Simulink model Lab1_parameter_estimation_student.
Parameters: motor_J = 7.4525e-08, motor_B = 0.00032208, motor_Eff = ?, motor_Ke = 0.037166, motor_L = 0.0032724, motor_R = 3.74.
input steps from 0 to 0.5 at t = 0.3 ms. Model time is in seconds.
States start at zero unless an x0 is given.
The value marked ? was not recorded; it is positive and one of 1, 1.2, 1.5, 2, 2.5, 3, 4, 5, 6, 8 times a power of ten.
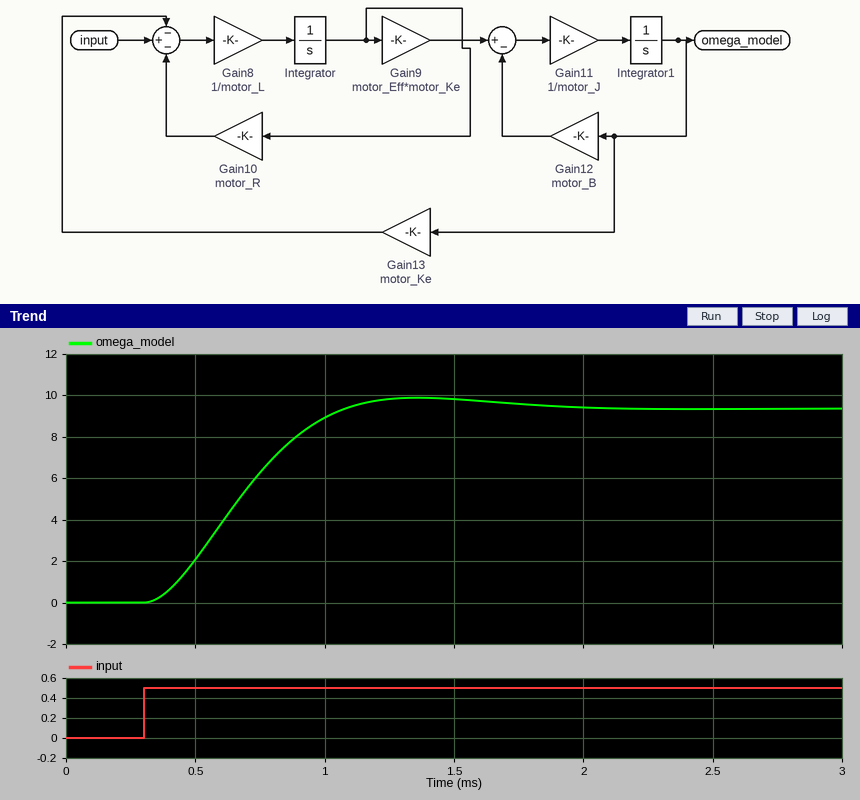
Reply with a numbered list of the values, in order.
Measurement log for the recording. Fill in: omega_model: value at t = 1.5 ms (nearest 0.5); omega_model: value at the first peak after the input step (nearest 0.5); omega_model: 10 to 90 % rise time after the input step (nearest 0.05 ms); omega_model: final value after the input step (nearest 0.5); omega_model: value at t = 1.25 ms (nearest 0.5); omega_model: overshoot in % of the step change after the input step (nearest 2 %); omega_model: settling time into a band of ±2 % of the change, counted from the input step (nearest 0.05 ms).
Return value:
1. 10.0
2. 10.0
3. 0.50 ms
4. 9.5
5. 10.0
6. 6 %
7. 1.50 ms
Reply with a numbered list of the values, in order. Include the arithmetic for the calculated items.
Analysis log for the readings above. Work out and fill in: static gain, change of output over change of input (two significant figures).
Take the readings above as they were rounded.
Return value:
1. (9.5 - 0) / (0.5 - 0) = 19
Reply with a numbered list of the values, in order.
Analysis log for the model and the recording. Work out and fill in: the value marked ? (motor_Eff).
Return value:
1. 2
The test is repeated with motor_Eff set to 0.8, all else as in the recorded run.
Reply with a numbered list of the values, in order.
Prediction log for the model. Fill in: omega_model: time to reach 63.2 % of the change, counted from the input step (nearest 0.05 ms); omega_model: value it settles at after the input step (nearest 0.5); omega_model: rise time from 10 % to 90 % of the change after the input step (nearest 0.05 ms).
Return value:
1. 0.65 ms
2. 6.5
3. 0.90 ms
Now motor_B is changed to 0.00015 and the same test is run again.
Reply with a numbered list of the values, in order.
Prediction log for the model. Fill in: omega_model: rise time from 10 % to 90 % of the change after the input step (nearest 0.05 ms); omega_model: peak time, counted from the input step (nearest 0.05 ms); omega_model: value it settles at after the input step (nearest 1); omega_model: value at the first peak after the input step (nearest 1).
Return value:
1. 0.40 ms
2. 0.95 ms
3. 11
4. 14
